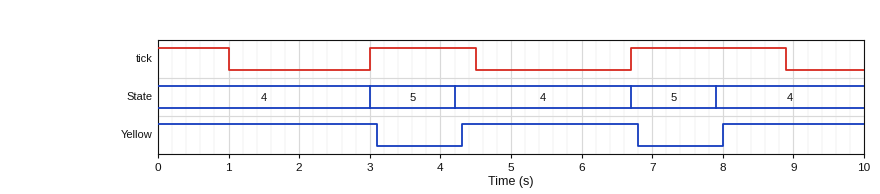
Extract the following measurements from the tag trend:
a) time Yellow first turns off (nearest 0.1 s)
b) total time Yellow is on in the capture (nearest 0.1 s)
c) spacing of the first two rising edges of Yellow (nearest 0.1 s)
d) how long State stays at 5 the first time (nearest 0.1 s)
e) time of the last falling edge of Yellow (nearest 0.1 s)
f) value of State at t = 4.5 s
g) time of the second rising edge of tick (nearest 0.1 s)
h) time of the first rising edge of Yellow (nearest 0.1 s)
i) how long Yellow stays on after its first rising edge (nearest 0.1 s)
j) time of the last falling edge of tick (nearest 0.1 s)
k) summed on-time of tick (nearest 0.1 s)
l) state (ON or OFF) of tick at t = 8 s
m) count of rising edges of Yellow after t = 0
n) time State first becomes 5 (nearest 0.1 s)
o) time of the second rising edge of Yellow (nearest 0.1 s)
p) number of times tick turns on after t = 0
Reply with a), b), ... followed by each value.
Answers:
a) 3.1 s
b) 7.6 s
c) 3.7 s
d) 1.2 s
e) 6.8 s
f) 4
g) 6.7 s
h) 4.3 s
i) 2.5 s
j) 8.9 s
k) 4.7 s
l) ON
m) 2
n) 3.0 s
o) 8.0 s
p) 2
